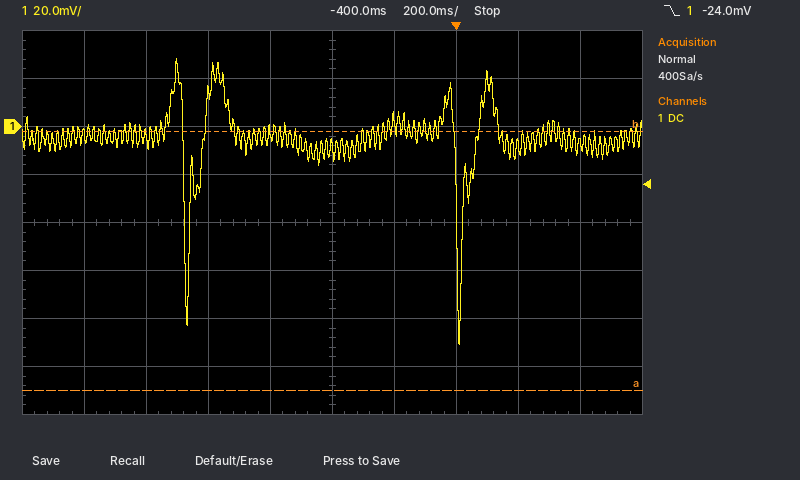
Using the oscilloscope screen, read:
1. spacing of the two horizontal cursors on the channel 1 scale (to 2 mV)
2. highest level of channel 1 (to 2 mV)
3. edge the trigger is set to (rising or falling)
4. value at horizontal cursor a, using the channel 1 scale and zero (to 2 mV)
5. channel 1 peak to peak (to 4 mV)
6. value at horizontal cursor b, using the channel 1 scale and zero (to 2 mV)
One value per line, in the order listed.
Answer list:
108 mV
28 mV
falling
-110 mV
120 mV
-2 mV
